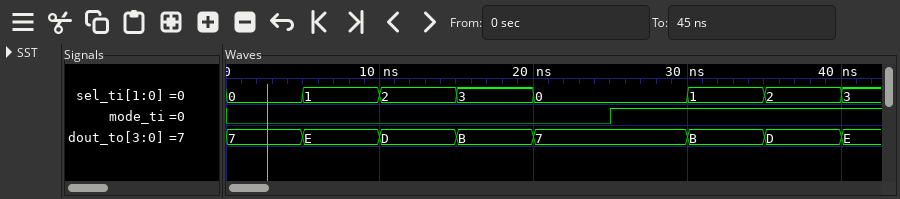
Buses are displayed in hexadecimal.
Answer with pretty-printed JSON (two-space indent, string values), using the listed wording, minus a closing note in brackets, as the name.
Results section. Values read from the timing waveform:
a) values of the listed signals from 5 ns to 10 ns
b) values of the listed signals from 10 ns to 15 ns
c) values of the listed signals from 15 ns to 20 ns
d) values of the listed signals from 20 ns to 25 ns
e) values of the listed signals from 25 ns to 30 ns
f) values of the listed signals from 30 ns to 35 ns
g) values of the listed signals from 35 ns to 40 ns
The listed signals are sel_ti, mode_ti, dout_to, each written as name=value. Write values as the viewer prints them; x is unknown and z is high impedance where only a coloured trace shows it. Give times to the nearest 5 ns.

{
  "values of the listed signals from 5 ns to 10 ns": "sel_ti=1, mode_ti=0, dout_to=E",
  "values of the listed signals from 10 ns to 15 ns": "sel_ti=2, mode_ti=0, dout_to=D",
  "values of the listed signals from 15 ns to 20 ns": "sel_ti=3, mode_ti=0, dout_to=B",
  "values of the listed signals from 20 ns to 25 ns": "sel_ti=0, mode_ti=0, dout_to=7",
  "values of the listed signals from 25 ns to 30 ns": "sel_ti=0, mode_ti=1, dout_to=7",
  "values of the listed signals from 30 ns to 35 ns": "sel_ti=1, mode_ti=1, dout_to=B",
  "values of the listed signals from 35 ns to 40 ns": "sel_ti=2, mode_ti=1, dout_to=D"
}
